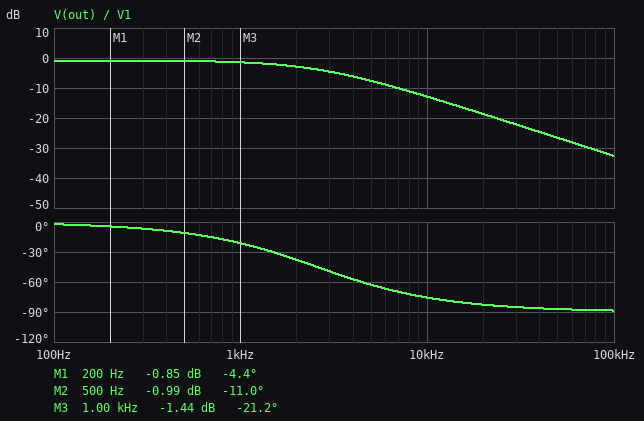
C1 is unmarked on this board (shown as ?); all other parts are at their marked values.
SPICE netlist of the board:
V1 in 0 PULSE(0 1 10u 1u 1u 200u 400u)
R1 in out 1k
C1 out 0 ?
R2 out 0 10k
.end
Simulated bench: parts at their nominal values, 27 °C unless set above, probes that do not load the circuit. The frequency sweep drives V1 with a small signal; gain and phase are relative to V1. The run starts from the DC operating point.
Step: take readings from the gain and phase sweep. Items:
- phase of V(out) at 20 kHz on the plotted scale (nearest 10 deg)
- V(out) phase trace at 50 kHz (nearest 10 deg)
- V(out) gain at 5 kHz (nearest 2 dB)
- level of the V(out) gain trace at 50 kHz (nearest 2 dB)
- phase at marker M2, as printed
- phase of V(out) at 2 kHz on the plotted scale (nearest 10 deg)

-80 deg
-90 deg
-8 dB
-26 dB
-11.0 deg
-40 deg
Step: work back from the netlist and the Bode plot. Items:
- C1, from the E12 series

68 nF
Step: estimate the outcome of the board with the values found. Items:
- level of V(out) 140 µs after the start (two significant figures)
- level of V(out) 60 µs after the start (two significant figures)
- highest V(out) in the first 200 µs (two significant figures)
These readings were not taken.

800 mV
500 mV
870 mV
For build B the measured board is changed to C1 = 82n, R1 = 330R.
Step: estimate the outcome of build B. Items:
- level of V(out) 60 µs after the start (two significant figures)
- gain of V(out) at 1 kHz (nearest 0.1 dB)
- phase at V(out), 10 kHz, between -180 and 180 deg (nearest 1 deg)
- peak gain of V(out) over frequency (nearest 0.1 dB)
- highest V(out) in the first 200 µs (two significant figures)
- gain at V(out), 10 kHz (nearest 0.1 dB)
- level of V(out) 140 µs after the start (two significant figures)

820 mV
-0.4 dB
-59 deg
-0.3 dB
970 mV
-6.0 dB
960 mV
